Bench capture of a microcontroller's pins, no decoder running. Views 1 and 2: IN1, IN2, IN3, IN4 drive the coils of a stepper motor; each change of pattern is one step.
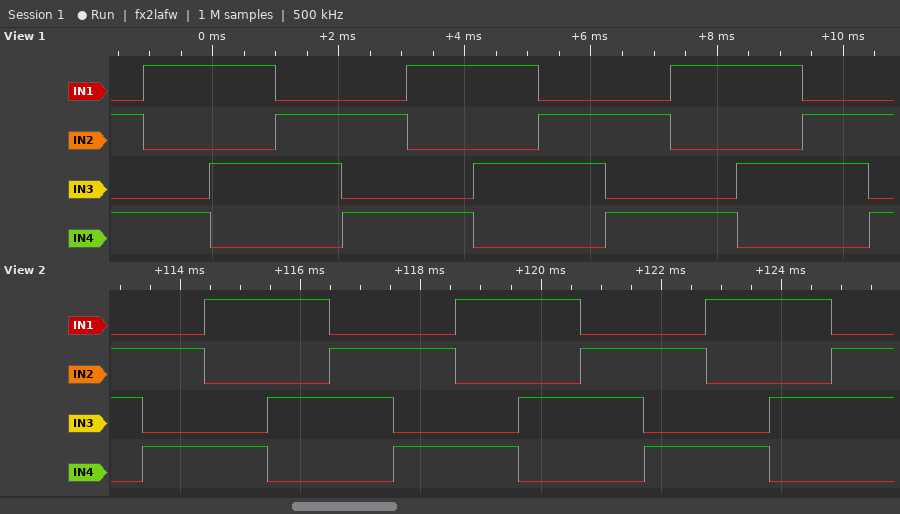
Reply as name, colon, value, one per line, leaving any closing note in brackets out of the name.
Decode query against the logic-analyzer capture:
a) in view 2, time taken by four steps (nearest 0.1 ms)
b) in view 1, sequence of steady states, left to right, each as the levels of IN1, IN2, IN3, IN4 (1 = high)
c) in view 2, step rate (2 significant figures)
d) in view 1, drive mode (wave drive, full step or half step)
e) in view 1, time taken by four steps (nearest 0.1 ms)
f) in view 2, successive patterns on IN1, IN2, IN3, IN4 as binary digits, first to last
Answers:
in view 2, time taken by four steps: 4.2 ms
in view 1, sequence of steady states, left to right, each as the levels of IN1, IN2, IN3, IN4: 0101 1001 1010 0110 0101 1001 1010 0110 0101 1001 1010 0110 0101
in view 2, step rate: 960 steps/s
in view 1, drive mode: full step
in view 1, time taken by four steps: 4.2 ms
in view 2, successive patterns on IN1, IN2, IN3, IN4 as binary digits, first to last: 0110 0101 1001 1010 0110 0101 1001 1010 0110 0101 1001 1010 0110
